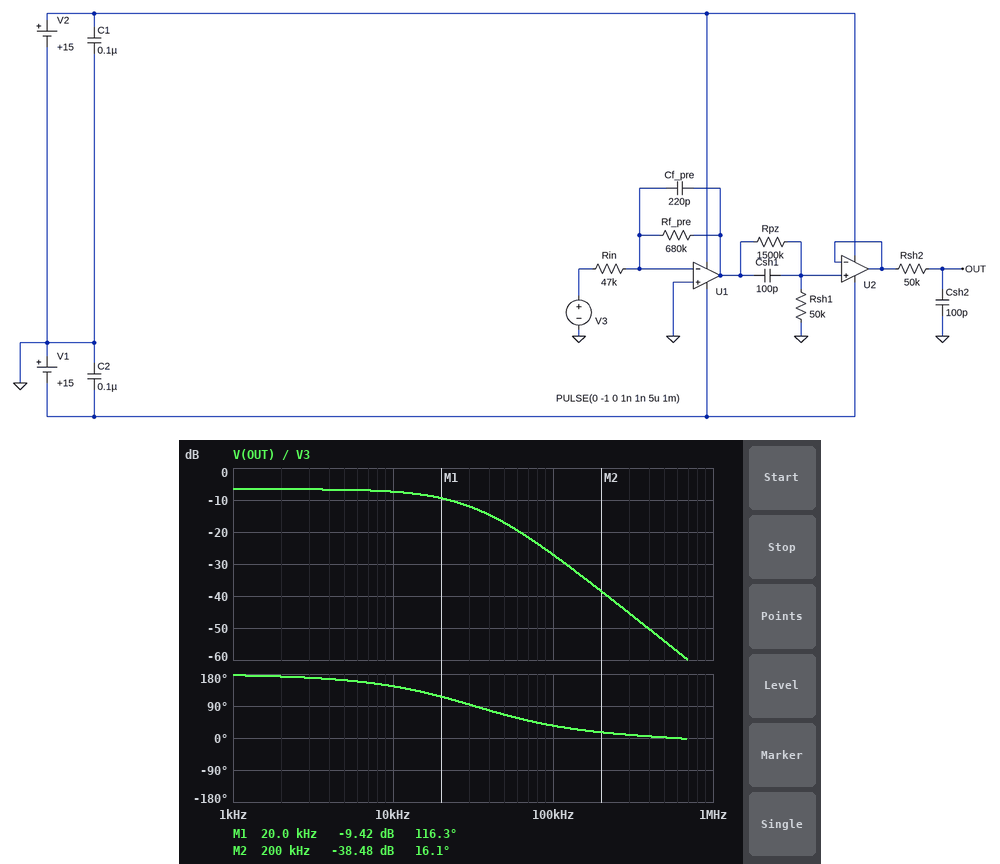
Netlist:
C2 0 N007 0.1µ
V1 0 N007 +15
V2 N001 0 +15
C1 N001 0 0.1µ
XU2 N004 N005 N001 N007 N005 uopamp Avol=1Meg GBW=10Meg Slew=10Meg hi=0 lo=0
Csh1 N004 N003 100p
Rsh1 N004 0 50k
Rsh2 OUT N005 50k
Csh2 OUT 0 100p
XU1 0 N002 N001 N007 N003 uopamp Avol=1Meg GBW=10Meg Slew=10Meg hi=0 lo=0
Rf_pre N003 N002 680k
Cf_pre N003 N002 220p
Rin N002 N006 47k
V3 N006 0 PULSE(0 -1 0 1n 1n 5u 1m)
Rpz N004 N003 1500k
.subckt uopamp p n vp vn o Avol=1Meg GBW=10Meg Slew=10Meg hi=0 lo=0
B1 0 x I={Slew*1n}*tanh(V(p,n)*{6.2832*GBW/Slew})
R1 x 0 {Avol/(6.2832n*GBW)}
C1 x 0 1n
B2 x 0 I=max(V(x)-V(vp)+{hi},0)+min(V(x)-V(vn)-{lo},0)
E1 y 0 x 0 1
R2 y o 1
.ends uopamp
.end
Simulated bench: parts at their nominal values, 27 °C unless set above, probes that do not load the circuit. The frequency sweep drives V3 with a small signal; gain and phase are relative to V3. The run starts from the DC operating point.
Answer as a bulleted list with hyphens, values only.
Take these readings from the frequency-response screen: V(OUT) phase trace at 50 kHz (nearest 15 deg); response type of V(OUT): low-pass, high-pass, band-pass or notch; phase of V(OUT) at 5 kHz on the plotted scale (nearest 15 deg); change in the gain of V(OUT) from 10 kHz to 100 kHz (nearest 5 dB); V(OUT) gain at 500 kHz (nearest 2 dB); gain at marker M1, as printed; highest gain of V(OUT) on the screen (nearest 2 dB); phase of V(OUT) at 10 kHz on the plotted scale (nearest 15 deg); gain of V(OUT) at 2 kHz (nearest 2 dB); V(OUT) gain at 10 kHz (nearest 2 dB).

- 60 deg
- low-pass
- 165 deg
- -20 dB
- -54 dB
- -9.42 dB
- -6 dB
- 150 deg
- -6 dB
- -8 dB
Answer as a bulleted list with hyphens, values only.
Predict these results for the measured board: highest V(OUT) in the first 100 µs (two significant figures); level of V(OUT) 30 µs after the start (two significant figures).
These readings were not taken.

- 170 mV
- 10 mV
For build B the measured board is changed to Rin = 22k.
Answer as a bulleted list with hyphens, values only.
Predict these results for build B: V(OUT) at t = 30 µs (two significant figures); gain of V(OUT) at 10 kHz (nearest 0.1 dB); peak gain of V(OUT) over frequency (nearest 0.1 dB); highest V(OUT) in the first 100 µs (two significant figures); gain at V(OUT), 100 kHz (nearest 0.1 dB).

- 22 mV
- -0.8 dB
- 0 dB
- 360 mV
- -20.5 dB
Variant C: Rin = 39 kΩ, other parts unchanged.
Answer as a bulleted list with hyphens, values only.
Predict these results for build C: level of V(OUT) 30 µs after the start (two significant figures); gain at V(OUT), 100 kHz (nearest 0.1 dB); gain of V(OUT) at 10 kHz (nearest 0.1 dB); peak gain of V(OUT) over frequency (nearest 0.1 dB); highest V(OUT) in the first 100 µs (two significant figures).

- 12 mV
- -25.5 dB
- -5.8 dB
- -5.0 dB
- 200 mV
